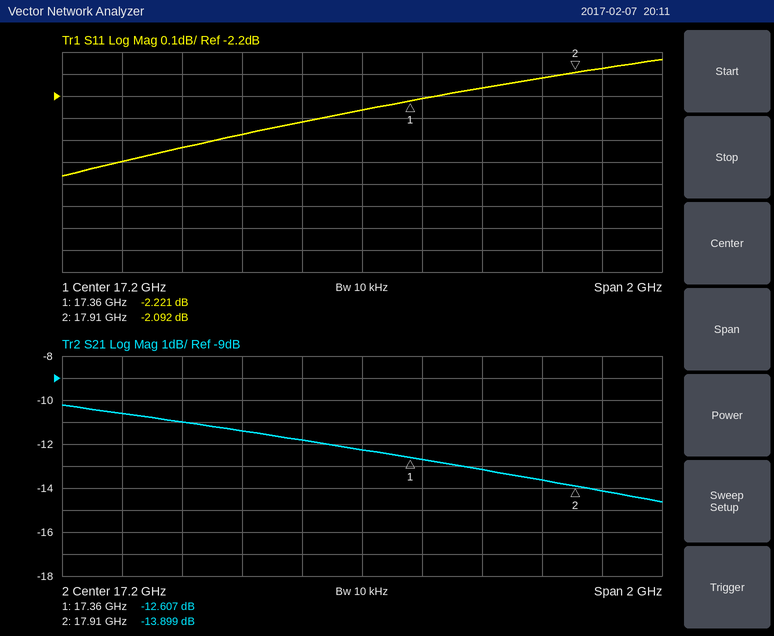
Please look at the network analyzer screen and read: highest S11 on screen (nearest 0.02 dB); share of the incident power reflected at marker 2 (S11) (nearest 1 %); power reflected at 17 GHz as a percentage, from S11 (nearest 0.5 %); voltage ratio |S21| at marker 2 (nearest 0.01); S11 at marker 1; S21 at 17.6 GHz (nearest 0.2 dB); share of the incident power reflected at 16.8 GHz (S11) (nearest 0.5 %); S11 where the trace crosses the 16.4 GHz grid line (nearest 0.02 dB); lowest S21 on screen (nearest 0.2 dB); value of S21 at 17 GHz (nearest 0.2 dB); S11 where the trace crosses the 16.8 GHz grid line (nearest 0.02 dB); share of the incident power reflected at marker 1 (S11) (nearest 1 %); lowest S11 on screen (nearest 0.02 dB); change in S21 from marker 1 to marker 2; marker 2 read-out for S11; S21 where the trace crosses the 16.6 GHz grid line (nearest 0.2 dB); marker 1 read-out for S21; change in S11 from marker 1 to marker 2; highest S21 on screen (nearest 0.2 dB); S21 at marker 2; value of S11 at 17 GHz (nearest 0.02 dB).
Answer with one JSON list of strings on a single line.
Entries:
["-2.04 dB", "62 %", "58.5 %", "0.20", "-2.221 dB", "-13.2 dB", "58.0 %", "-2.50 dB", "-14.6 dB", "-11.8 dB", "-2.38 dB", "60 %", "-2.56 dB", "-1.292 dB", "-2.092 dB", "-11.0 dB", "-12.607 dB", "0.129 dB", "-10.2 dB", "-13.899 dB", "-2.32 dB"]
